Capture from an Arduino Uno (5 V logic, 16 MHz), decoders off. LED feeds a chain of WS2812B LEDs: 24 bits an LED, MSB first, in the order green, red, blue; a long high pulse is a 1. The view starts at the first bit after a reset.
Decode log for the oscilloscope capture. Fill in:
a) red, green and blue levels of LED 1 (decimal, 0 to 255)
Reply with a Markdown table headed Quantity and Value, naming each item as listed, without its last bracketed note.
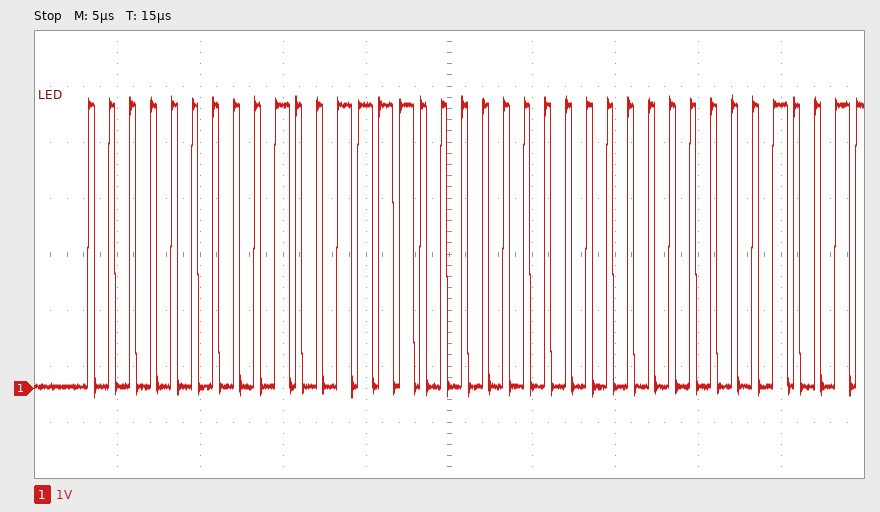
| Quantity | Value |
|---|---|
| red, green and blue levels of LED 1 | 79, 0, 0 |
